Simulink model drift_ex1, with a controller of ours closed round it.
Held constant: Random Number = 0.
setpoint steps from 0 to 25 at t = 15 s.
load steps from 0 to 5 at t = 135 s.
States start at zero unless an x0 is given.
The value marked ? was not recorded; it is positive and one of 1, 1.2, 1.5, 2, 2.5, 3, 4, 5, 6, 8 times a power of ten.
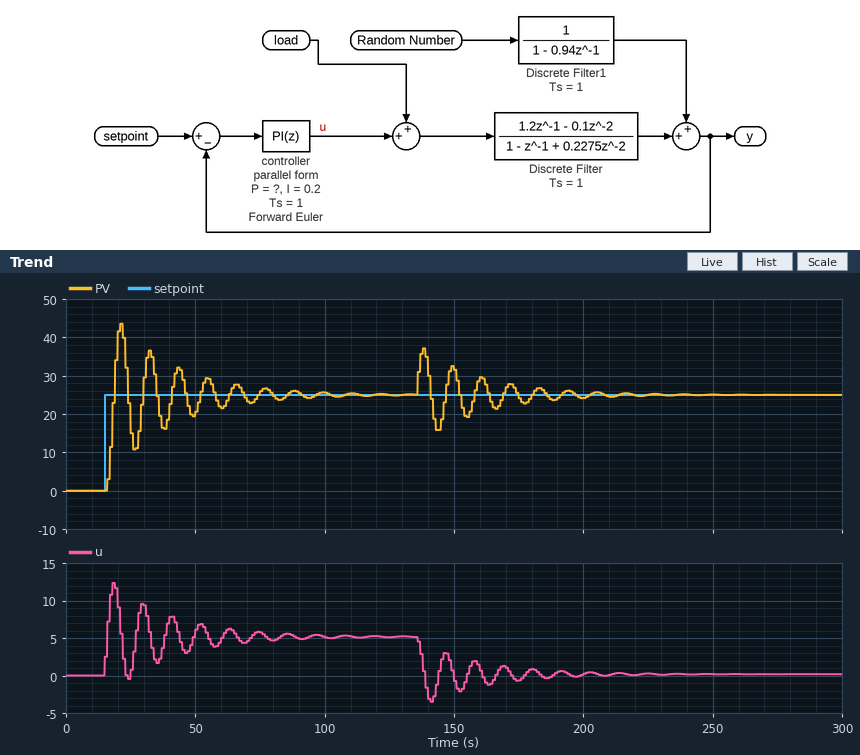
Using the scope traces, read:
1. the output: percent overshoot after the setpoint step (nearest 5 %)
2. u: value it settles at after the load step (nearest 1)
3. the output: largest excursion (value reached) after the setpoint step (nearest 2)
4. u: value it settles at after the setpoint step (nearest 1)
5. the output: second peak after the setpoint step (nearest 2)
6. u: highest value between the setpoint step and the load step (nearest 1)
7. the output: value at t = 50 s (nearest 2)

75 %
0
44
5
36
12
20
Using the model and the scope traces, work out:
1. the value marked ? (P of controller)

0.1
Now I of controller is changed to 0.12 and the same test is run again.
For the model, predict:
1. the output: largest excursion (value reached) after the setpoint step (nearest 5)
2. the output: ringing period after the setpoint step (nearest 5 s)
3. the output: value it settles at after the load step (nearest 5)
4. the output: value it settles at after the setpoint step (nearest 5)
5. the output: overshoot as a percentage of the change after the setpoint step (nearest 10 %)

35
15 s
25
25
40 %
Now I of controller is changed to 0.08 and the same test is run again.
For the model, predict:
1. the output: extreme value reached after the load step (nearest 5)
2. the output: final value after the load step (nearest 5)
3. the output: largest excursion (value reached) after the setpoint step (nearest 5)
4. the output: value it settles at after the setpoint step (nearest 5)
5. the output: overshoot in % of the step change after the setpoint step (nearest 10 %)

40
25
30
25
20 %
